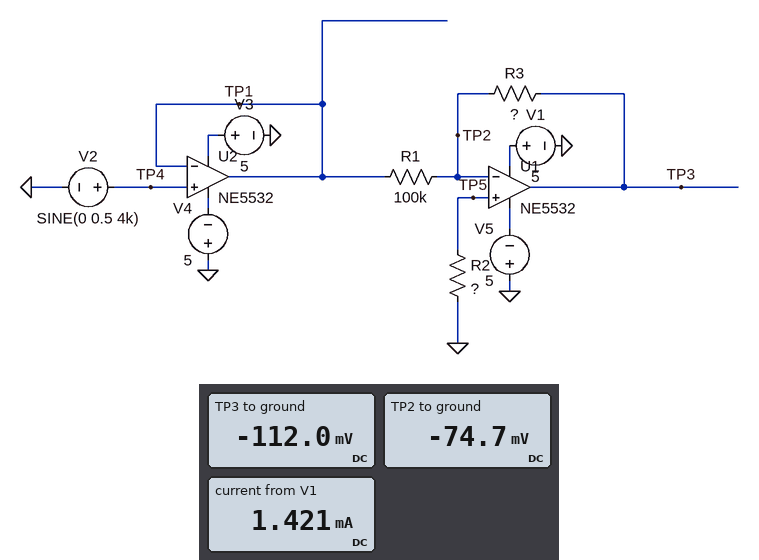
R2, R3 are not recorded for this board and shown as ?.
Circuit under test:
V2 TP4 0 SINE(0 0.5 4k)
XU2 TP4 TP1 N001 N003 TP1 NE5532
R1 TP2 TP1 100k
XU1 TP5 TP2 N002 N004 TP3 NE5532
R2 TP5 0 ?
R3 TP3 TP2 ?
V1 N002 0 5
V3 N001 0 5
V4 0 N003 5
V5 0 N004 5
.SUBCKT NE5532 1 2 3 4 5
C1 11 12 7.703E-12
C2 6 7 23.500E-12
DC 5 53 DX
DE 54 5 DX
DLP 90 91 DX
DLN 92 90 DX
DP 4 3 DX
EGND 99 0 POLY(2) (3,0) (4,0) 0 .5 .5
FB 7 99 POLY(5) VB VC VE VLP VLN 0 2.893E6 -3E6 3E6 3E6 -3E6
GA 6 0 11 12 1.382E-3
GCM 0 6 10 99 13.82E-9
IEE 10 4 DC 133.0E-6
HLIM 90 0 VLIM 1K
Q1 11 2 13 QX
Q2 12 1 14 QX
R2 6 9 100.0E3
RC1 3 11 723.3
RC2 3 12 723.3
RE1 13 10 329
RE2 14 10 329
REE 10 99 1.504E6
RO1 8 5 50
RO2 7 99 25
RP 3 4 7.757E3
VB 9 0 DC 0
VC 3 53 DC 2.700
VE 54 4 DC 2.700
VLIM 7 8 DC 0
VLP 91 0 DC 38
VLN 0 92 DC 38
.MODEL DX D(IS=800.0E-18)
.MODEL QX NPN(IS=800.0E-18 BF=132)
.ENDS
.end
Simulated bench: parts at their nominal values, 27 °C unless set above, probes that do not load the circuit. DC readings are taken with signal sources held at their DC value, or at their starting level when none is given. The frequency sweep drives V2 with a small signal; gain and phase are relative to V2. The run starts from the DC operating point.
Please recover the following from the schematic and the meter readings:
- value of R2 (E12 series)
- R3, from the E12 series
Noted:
150 kΩ
150 kΩ
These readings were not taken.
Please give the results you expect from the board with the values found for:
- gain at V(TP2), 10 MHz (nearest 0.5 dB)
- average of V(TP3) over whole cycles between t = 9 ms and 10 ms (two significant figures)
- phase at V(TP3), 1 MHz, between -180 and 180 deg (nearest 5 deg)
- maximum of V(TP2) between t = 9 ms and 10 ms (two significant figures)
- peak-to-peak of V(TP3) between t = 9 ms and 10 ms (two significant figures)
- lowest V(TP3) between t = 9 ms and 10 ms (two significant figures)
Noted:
-6.0 dB
-110 mV
145 deg
-74 mV
1.5 V
-860 mV
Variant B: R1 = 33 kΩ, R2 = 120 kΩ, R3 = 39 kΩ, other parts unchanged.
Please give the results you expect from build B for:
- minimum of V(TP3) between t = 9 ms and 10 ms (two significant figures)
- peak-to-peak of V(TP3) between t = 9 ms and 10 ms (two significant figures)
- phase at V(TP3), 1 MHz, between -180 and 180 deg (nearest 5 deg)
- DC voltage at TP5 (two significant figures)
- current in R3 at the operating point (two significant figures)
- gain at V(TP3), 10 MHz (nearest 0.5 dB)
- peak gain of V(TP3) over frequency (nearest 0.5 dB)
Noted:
-700 mV
1.2 V
150 deg
-60 mV
1.3 µA
-12.5 dB
1.5 dB
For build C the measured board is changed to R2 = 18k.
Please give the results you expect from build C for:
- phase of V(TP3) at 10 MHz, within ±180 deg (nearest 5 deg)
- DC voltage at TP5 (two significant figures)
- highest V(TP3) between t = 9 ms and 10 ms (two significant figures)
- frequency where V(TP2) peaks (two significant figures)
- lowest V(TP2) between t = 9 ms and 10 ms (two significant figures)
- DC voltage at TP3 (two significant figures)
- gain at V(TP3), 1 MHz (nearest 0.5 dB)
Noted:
-10 deg
-9.0 mV
800 mV
7.0 MHz
-9.3 mV
52 mV
3.0 dB
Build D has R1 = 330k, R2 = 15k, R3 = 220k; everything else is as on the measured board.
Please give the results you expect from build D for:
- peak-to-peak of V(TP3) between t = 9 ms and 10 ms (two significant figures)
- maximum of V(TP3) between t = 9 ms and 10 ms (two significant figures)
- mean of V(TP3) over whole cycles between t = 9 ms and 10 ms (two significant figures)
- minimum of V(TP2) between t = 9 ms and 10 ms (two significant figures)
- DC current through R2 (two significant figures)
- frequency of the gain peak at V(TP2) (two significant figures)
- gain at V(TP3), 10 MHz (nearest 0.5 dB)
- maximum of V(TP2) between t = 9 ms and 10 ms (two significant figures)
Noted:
670 mV
430 mV
97 mV
-7.6 mV
500 nA
7.3 MHz
-15.0 dB
-7.3 mV
